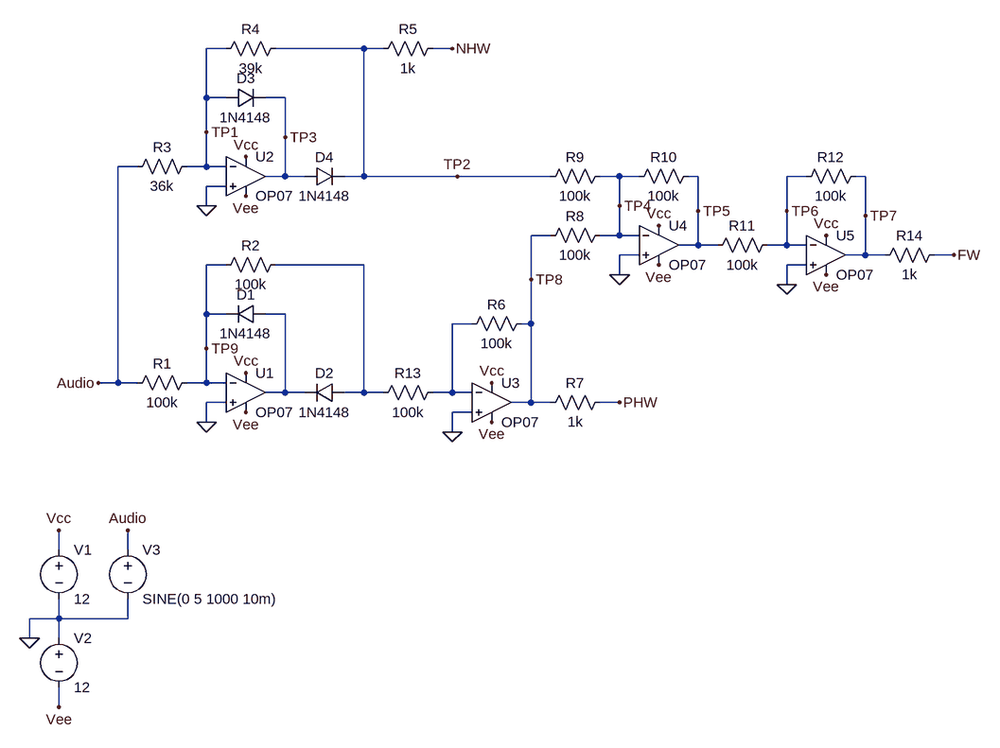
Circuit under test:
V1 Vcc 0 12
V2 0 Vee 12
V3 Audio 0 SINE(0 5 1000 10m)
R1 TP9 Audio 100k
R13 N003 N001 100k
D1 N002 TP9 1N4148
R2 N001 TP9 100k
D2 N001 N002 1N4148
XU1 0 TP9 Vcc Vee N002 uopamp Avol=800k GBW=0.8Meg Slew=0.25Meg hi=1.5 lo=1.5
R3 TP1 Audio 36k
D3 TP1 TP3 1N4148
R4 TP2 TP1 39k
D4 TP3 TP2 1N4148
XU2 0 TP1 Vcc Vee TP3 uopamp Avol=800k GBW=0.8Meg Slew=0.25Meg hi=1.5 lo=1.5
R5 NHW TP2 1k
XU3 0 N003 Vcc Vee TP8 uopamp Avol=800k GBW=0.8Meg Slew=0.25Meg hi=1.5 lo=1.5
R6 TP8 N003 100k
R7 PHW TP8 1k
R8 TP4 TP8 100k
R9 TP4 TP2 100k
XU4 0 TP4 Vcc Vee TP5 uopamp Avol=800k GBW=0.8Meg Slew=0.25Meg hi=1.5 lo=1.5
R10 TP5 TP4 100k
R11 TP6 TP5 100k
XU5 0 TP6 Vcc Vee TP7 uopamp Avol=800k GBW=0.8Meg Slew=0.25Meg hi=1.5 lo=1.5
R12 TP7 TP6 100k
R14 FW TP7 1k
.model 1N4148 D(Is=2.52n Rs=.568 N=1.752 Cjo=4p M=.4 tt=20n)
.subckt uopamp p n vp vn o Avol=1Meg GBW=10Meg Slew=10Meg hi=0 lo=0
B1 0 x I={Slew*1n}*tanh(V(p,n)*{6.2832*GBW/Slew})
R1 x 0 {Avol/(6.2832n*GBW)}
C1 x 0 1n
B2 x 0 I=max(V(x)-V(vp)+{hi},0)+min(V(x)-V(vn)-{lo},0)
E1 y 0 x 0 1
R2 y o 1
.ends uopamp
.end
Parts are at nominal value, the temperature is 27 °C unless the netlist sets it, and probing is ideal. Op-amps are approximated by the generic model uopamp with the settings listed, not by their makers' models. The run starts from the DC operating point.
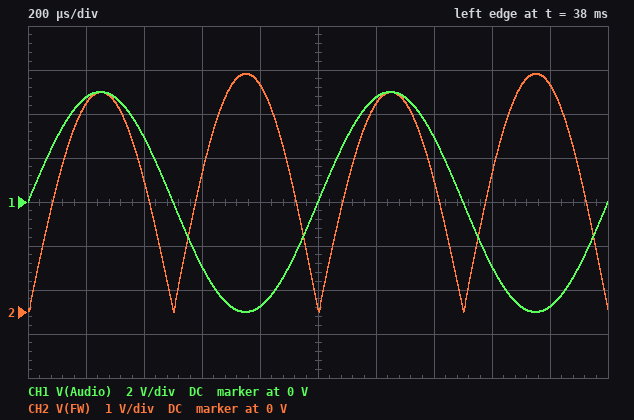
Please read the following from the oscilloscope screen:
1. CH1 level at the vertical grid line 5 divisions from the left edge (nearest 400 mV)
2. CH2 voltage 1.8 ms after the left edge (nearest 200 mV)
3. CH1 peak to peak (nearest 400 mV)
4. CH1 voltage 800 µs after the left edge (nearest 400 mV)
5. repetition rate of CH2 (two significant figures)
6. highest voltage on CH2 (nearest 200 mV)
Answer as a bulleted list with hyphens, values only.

- 0 V
- 5.2 V
- 10.0 V
- -4.8 V
- 2.0 kHz
- 5.4 V
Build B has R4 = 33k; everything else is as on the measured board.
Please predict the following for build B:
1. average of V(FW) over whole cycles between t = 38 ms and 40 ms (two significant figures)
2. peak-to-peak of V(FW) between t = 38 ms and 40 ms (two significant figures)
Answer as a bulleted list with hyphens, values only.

- 3.1 V
- 5.0 V
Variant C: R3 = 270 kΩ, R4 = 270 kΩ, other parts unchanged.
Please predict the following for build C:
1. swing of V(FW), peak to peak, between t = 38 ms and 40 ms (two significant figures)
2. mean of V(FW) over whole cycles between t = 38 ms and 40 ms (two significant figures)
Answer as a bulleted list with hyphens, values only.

- 5.0 V
- 3.2 V
